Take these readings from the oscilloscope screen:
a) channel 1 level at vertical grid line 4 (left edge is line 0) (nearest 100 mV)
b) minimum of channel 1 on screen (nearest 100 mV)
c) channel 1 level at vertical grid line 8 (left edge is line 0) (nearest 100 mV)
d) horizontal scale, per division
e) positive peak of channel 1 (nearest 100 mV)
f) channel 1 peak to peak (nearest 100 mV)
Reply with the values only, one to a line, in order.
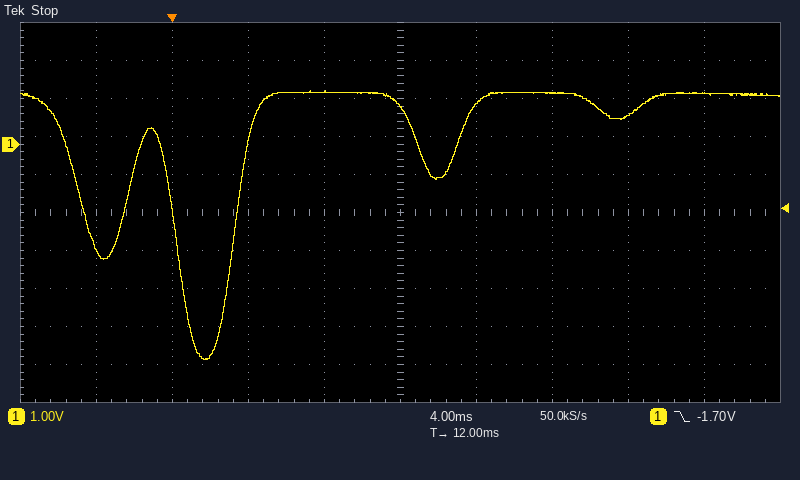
1.4 V
-5.7 V
700 mV
4 ms
1.4 V
7.1 V
